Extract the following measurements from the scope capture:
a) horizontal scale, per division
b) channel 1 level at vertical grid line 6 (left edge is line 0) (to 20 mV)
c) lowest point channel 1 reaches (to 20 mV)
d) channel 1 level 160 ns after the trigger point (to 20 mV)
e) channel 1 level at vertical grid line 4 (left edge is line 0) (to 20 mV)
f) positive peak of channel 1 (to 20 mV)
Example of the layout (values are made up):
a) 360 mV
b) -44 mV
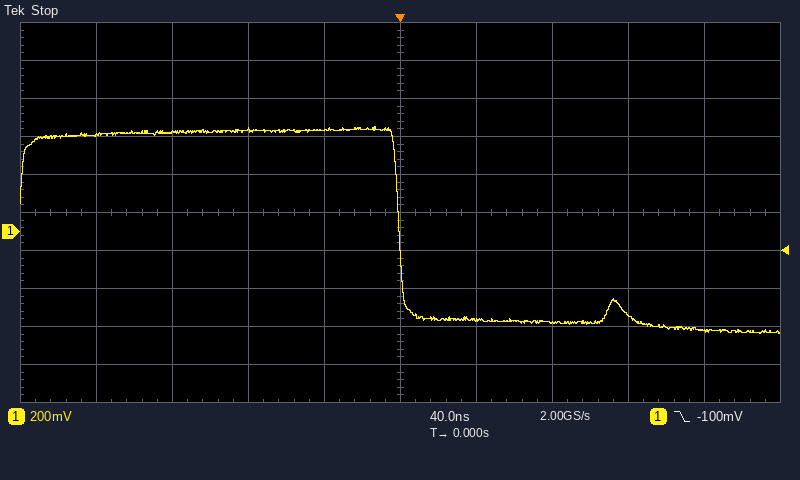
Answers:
a) 40 ns
b) -460 mV
c) -540 mV
d) -520 mV
e) 540 mV
f) 560 mV
